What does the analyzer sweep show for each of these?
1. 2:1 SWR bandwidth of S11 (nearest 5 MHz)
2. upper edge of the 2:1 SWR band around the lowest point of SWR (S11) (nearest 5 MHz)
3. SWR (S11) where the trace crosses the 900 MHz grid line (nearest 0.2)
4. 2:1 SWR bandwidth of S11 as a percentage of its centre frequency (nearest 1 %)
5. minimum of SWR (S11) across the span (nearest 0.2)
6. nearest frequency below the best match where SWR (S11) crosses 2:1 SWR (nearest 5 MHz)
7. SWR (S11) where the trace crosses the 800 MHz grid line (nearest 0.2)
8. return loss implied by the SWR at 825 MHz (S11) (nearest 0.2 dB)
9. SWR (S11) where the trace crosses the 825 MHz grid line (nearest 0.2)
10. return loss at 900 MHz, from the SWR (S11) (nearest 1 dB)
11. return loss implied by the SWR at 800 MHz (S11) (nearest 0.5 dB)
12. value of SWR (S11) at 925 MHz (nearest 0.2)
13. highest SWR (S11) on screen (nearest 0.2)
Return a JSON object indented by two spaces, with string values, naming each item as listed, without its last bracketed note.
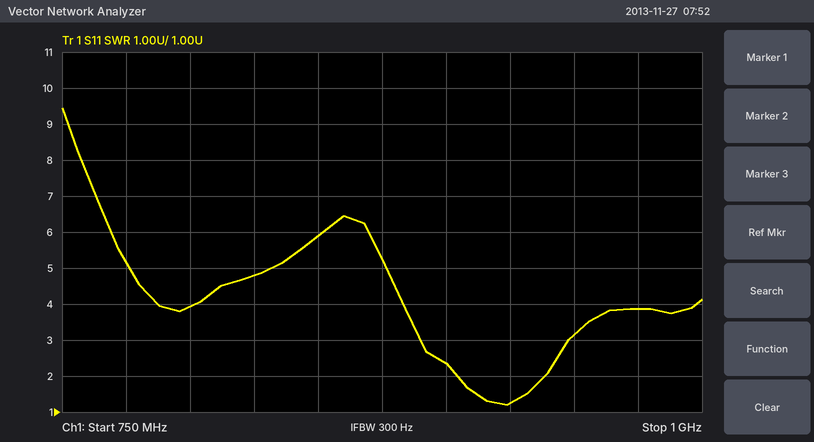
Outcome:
{
  "2:1 SWR bandwidth of S11": "35 MHz",
  "upper edge of the 2:1 SWR band around the lowest point of SWR (S11)": "940 MHz",
  "SWR (S11) where the trace crosses the 900 MHz grid line": "2.4",
  "2:1 SWR bandwidth of S11 as a percentage of its centre frequency": "4 %",
  "minimum of SWR (S11) across the span": "1.2",
  "nearest frequency below the best match where SWR (S11) crosses 2:1 SWR": "905 MHz",
  "SWR (S11) where the trace crosses the 800 MHz grid line": "4.0",
  "return loss implied by the SWR at 825 MHz (S11)": "3.6 dB",
  "SWR (S11) where the trace crosses the 825 MHz grid line": "4.8",
  "return loss at 900 MHz, from the SWR (S11)": "8 dB",
  "return loss implied by the SWR at 800 MHz (S11)": "4.5 dB",
  "value of SWR (S11) at 925 MHz": "1.2",
  "highest SWR (S11) on screen": "9.4"
}
